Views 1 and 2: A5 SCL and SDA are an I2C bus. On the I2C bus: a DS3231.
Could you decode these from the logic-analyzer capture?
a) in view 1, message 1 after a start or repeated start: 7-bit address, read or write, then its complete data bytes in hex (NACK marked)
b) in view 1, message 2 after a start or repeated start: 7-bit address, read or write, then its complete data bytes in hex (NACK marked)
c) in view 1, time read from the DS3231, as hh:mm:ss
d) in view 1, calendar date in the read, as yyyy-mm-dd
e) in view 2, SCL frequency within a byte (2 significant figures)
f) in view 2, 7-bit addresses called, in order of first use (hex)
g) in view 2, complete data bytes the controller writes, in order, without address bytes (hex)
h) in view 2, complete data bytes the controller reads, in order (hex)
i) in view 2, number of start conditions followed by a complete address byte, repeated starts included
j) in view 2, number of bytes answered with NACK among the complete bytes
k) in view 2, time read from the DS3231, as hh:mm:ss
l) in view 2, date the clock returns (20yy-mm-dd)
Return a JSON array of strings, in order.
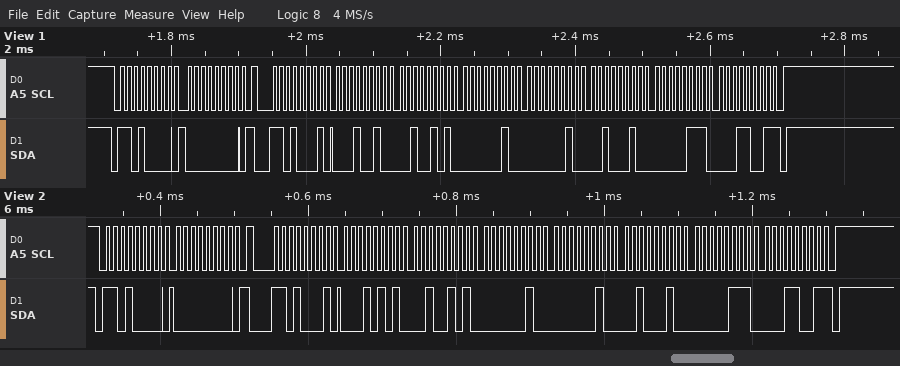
["0x68 write: 00", "0x68 read: 12 25 02 02 22 07 19 NACK", "02:25:12", "2019-07-22", "100 kHz", "0x68", "00", "15 25 02 02 22 07 19", "2", "1", "02:25:15", "2019-07-22"]
